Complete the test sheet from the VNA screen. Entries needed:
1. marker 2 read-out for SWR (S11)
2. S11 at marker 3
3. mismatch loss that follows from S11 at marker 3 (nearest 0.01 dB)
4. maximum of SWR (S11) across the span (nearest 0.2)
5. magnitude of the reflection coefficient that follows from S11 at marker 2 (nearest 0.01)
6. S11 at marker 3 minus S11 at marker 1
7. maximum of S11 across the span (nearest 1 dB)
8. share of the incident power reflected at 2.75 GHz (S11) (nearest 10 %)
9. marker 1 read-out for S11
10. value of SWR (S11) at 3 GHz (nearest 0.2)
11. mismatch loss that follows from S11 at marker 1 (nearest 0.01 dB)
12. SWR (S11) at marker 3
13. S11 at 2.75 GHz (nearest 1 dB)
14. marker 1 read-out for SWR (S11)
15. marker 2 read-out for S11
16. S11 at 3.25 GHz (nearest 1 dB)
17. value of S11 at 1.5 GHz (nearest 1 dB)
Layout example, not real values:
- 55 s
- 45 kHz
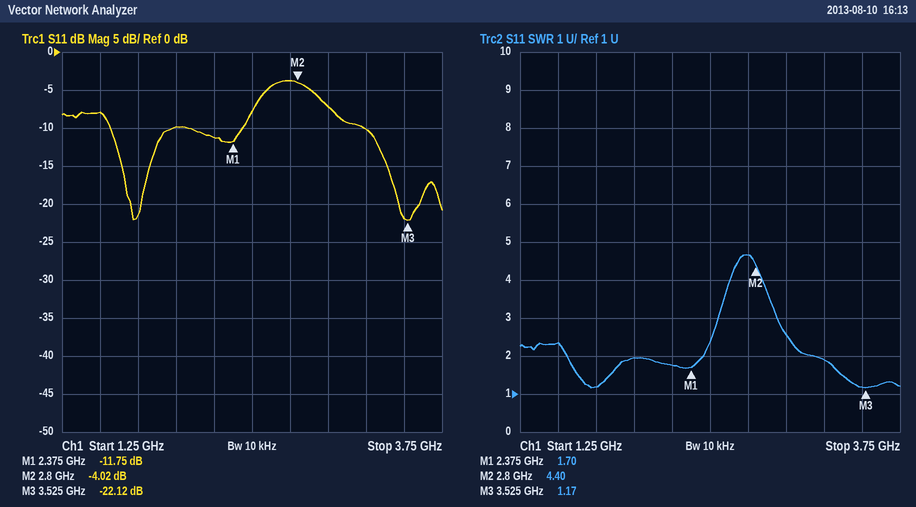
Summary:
- 4.40
- -22.12 dB
- 0.03 dB
- 4.6
- 0.63
- -10.37 dB
- -4 dB
- 40 %
- -11.75 dB
- 2.6
- 0.30 dB
- 1.17
- -4 dB
- 1.70
- -4.02 dB
- -10 dB
- -8 dB
